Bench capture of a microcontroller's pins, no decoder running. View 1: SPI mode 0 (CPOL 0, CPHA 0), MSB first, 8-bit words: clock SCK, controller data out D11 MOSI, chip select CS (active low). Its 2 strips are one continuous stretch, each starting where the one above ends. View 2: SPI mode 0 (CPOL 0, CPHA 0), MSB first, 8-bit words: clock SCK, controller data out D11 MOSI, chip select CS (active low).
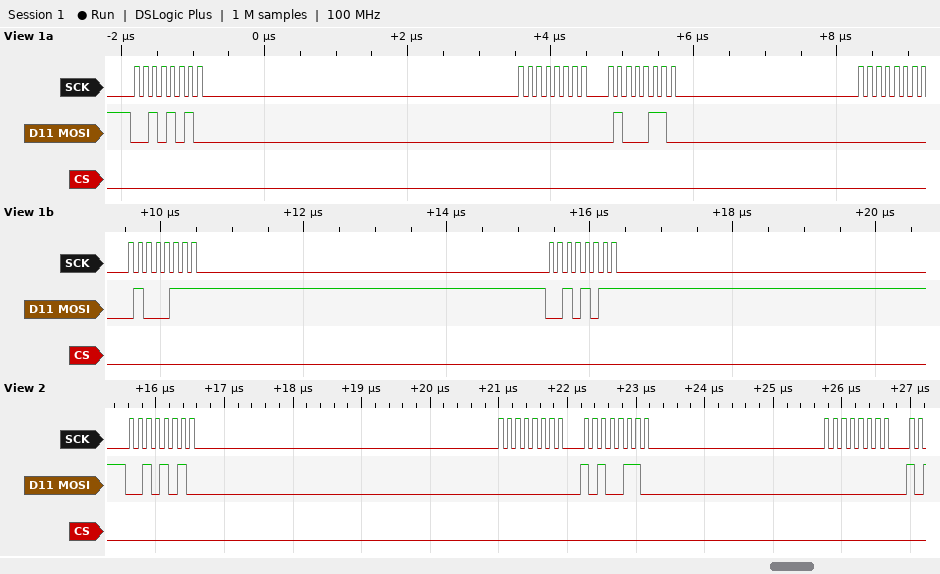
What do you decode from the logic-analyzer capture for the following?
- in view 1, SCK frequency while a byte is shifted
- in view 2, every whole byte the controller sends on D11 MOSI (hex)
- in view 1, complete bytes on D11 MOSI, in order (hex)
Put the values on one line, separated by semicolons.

8 MHz; 2A 00 A6 00; 2A 00 46 00 47 2B
